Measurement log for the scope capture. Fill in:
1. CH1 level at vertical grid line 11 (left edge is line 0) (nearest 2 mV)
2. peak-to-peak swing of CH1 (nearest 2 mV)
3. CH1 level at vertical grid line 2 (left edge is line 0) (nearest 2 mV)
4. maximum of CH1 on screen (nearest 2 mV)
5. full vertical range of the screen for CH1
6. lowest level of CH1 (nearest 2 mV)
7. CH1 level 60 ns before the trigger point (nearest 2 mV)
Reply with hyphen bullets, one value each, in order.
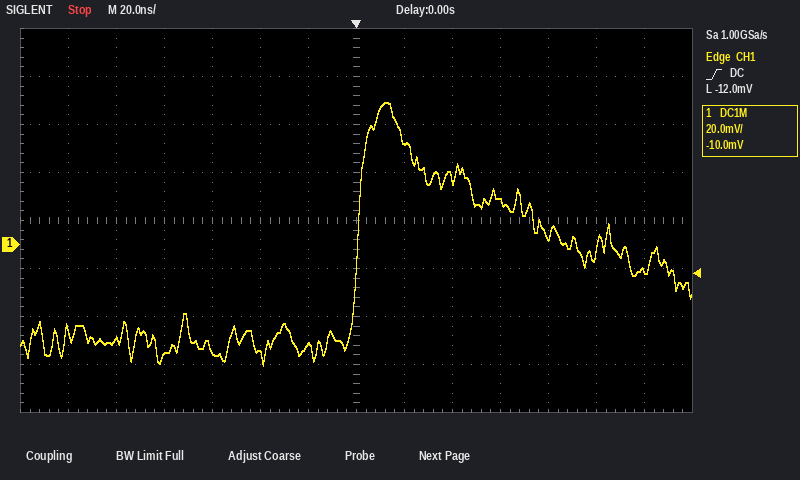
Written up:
- 2 mV
- 110 mV
- -40 mV
- 60 mV
- 160 mV
- -50 mV
- -44 mV
